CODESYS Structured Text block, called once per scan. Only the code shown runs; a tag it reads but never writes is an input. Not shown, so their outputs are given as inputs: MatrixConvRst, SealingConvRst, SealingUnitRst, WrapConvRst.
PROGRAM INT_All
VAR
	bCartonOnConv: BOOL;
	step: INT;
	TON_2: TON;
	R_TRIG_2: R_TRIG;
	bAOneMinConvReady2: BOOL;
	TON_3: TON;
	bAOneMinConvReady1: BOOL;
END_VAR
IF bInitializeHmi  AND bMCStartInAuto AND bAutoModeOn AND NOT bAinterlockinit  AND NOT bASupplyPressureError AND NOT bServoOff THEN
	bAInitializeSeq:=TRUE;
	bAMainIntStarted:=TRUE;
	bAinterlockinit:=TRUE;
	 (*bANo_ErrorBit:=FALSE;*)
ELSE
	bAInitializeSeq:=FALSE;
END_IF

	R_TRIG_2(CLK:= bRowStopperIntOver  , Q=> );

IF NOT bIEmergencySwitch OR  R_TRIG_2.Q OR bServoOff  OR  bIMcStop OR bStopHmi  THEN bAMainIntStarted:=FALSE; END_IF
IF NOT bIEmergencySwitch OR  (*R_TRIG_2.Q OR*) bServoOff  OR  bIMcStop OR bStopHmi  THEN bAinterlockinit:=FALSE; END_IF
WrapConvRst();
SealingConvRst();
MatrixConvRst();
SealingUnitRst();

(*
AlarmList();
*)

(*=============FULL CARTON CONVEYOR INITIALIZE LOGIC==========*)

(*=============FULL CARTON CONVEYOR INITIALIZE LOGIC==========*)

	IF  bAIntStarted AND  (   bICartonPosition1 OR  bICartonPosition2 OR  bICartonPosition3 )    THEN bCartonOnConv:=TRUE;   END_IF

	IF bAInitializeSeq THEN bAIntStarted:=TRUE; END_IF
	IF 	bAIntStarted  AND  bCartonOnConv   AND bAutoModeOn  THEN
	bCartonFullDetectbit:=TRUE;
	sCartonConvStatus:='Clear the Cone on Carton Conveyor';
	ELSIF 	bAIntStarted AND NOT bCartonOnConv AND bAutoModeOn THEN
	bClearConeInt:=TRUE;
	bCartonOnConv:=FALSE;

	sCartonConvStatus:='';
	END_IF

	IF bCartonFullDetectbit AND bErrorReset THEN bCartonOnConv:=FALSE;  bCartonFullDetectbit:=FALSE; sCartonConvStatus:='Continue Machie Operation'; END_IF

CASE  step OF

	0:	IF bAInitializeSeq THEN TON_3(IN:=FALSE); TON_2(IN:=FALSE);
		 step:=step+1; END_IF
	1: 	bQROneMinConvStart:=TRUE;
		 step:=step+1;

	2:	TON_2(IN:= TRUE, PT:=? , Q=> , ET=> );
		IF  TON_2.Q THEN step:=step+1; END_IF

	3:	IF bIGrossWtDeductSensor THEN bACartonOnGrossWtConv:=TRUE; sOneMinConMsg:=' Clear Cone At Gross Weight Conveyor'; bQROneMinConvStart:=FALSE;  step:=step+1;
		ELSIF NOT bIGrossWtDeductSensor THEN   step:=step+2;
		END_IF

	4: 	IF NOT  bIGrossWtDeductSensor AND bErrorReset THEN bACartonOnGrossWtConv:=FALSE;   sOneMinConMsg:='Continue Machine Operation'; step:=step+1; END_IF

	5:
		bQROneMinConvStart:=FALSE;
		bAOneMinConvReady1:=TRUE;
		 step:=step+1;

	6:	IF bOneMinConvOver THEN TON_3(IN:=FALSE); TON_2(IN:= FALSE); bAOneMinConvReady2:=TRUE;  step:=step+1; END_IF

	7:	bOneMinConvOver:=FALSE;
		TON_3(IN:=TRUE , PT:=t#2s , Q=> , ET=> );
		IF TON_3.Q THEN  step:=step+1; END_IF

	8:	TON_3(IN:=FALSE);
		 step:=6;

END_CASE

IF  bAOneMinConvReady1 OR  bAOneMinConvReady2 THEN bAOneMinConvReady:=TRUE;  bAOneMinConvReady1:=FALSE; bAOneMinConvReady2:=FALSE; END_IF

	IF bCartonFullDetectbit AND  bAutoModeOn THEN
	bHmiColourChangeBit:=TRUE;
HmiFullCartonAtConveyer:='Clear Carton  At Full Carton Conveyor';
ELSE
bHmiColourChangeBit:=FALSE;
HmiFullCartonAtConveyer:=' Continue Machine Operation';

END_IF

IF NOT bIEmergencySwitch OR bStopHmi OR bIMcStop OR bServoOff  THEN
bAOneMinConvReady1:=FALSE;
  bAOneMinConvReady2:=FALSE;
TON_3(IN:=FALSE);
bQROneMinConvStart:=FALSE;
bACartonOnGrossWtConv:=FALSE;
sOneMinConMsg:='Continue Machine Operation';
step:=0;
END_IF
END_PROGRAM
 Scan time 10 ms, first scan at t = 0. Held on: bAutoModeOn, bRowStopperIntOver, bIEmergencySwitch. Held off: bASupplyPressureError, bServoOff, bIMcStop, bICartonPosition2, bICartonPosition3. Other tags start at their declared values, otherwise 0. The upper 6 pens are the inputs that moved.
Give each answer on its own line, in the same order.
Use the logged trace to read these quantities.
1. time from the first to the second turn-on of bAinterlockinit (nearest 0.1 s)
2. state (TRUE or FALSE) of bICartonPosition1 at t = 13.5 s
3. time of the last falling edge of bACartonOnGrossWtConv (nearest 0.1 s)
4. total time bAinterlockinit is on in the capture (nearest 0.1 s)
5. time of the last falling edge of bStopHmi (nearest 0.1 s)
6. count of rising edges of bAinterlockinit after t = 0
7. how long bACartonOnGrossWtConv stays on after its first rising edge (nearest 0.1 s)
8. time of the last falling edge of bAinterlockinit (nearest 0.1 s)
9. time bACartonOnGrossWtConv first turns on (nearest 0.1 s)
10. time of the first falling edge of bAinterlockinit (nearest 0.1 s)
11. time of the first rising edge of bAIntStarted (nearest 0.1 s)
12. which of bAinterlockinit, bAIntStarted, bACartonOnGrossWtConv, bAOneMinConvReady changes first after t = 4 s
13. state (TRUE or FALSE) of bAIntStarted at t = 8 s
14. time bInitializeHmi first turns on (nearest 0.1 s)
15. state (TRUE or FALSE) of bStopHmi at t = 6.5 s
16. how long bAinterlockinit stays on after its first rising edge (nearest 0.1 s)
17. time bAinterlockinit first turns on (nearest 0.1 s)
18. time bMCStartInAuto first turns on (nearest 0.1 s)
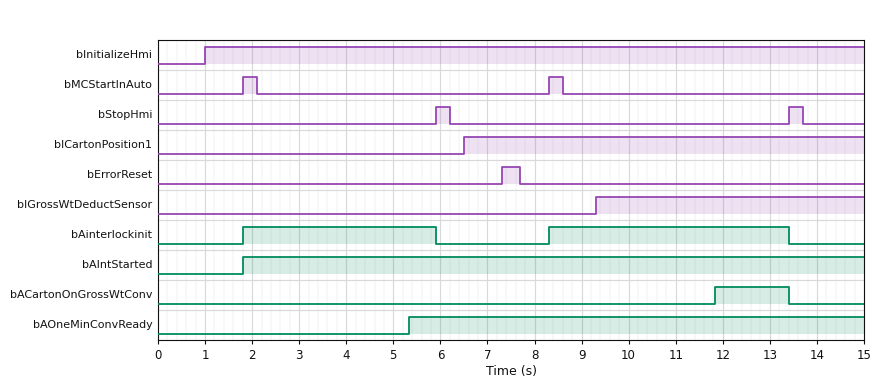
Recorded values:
6.5 s
TRUE
13.4 s
9.2 s
13.7 s
2
1.6 s
13.4 s
11.8 s
5.9 s
1.8 s
bAOneMinConvReady
TRUE
1.0 s
FALSE
4.1 s
1.8 s
1.8 s
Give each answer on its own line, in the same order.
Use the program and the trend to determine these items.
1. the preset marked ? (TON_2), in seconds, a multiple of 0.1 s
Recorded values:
3.5 s
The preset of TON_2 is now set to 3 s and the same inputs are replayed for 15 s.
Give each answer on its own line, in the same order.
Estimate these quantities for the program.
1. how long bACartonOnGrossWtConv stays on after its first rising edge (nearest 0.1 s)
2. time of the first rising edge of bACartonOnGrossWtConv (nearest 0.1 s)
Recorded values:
2.1 s
11.3 s
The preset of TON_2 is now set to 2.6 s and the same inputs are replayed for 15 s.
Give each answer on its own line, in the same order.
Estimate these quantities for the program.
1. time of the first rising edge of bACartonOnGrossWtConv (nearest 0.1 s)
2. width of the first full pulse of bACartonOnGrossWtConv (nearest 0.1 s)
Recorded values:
10.9 s
2.5 s
